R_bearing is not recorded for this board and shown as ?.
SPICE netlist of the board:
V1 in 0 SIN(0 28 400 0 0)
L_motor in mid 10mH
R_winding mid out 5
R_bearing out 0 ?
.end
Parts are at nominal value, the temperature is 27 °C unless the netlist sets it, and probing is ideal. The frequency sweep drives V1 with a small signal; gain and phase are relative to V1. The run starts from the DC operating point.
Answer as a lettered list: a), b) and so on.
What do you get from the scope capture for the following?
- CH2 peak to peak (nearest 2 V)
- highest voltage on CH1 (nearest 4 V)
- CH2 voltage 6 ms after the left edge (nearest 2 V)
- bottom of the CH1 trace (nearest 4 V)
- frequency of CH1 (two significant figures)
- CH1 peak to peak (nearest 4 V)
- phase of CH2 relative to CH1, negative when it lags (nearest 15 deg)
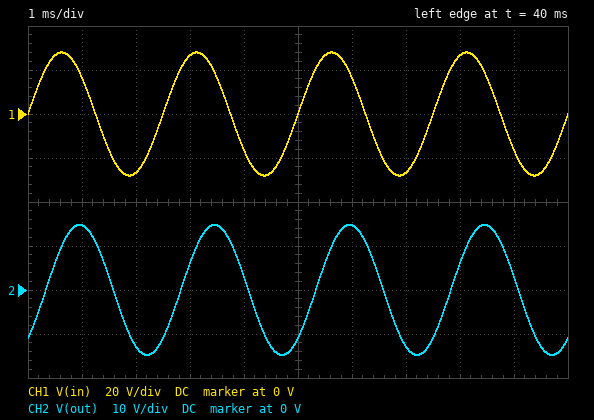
a) 30 V
b) 28 V
c) 14 V
d) -28 V
e) 400 Hz
f) 56 V
g) -45 deg
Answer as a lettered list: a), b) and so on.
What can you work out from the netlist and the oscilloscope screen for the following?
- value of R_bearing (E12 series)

a) 18 Ω
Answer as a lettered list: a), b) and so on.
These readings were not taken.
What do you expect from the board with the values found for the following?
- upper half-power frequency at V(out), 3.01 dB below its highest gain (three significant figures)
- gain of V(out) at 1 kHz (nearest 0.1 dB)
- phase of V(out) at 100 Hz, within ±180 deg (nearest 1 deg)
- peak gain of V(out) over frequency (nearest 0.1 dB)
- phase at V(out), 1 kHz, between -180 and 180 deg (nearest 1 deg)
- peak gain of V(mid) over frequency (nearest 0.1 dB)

a) 366 Hz
b) -11.4 dB
c) -15 deg
d) -2.1 dB
e) -70 deg
f) 0 dB
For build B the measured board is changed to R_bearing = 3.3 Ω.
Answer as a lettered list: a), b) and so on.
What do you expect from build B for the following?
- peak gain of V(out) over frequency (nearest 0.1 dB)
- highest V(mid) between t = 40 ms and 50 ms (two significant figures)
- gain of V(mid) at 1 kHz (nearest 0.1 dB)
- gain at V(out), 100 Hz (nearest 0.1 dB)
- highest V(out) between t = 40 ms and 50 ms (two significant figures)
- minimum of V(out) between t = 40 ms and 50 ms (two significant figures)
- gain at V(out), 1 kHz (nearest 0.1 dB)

a) -8.0 dB
b) 8.8 V
c) -17.7 dB
d) -10.0 dB
e) 3.5 V
f) -3.5 V
g) -25.7 dB
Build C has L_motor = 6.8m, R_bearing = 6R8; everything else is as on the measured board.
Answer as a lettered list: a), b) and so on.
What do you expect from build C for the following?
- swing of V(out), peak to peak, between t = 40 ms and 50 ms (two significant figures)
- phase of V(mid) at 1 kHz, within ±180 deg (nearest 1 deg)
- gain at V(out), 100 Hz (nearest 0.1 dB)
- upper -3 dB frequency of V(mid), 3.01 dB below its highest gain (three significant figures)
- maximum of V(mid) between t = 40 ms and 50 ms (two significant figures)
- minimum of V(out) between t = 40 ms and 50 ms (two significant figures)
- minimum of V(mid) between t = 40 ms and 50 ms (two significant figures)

a) 18 V
b) -75 deg
c) -5.3 dB
d) 276 Hz
e) 16 V
f) -9.2 V
g) -16 V
